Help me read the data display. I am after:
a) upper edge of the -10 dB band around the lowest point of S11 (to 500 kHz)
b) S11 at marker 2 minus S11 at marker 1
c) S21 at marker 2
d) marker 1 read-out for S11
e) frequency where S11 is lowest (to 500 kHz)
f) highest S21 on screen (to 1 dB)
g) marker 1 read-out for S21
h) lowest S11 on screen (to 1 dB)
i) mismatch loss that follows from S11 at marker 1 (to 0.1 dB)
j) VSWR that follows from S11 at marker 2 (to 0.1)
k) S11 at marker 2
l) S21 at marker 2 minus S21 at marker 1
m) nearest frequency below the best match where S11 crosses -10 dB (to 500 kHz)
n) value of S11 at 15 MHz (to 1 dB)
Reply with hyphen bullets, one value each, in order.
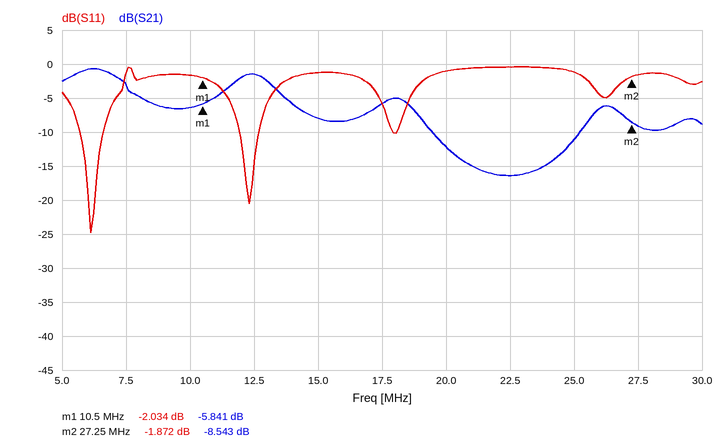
- 6.5 MHz
- 0.162 dB
- -8.543 dB
- -2.034 dB
- 6.0 MHz
- -1 dB
- -5.841 dB
- -25 dB
- 4.3 dB
- 9.3
- -1.872 dB
- -2.702 dB
- 5.5 MHz
- -1 dB
